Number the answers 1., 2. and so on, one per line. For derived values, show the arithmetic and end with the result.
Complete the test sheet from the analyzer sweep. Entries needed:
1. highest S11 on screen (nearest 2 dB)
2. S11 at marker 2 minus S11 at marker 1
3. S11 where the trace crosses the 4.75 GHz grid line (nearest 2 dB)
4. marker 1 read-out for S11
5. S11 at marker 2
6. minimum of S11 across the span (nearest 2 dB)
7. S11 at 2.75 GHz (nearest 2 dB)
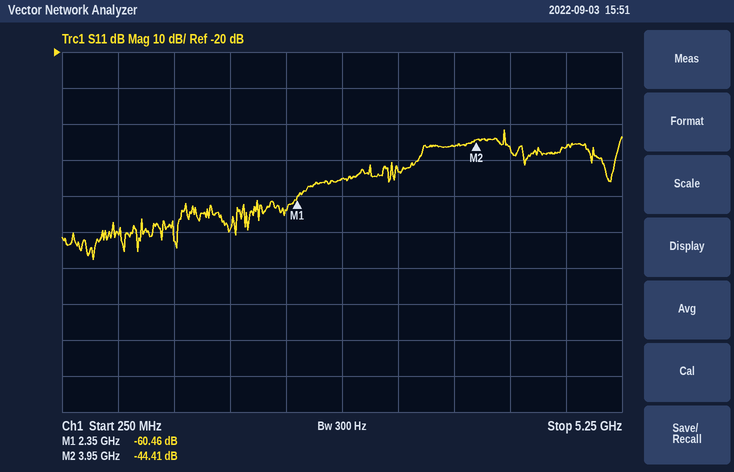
1. -42 dB
2. -44.41 − (-60.46) = 16.05 dB
3. -46 dB
4. -60.46 dB
5. -44.41 dB
6. -78 dB
7. -56 dB
